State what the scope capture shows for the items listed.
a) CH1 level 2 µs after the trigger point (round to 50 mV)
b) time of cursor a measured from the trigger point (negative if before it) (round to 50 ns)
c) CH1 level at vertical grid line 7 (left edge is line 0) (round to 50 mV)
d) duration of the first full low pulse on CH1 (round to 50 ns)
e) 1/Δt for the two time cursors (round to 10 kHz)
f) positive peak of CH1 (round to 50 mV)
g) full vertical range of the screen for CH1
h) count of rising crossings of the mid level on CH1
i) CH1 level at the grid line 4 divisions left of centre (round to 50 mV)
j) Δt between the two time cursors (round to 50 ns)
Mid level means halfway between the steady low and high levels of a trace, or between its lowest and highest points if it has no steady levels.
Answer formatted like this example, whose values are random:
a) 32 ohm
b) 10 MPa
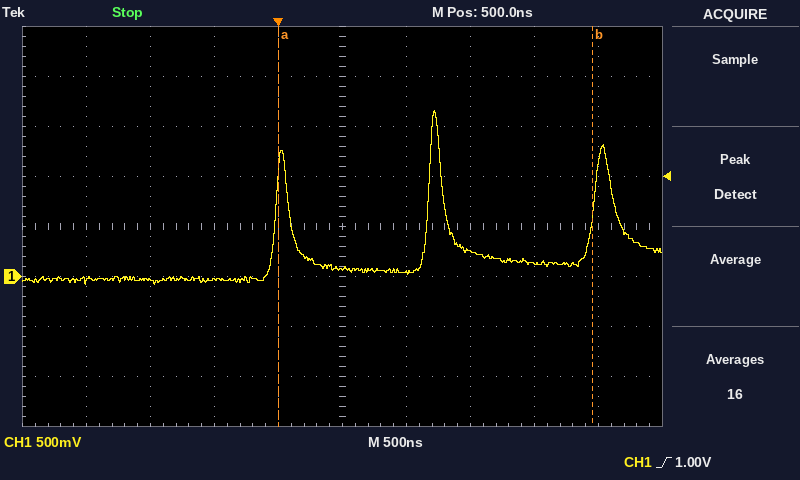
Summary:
a) 150 mV
b) 0 ns
c) 250 mV
d) 1.10 µs
e) 410 kHz
f) 1.65 V
g) 4 V
h) 3
i) -50 mV
j) 2.45 µs
